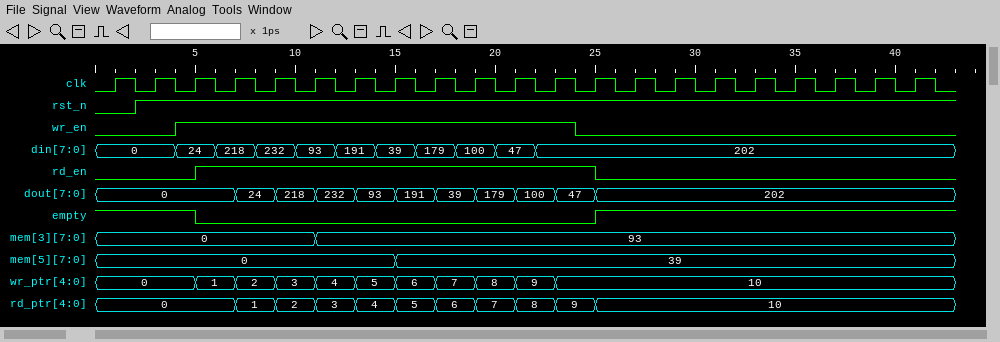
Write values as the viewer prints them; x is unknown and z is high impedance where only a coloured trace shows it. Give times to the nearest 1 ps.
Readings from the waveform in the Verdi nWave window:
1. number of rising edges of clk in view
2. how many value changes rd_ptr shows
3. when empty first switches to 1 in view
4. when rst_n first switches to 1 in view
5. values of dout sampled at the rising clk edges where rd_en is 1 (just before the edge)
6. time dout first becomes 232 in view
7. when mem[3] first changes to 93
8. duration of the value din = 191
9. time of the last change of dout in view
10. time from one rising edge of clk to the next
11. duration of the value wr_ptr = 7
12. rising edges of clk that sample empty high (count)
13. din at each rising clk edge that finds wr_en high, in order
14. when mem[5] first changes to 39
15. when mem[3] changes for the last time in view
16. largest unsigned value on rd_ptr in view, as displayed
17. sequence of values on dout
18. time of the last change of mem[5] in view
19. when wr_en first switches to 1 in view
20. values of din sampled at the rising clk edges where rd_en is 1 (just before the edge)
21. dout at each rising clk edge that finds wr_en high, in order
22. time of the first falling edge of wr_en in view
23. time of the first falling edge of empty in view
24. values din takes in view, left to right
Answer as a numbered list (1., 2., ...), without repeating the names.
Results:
1. 21
2. 10
3. 25 ps
4. 2 ps
5. 0, 24, 218, 232, 93, 191, 39, 179, 100, 47
6. 11 ps
7. 11 ps
8. 2 ps
9. 25 ps
10. 2 ps
11. 2 ps
12. 11
13. 24, 218, 232, 93, 191, 39, 179, 100, 47, 202
14. 15 ps
15. 11 ps
16. 10
17. 0, 24, 218, 232, 93, 191, 39, 179, 100, 47, 202
18. 15 ps
19. 4 ps
20. 218, 232, 93, 191, 39, 179, 100, 47, 202, 202
21. 0, 0, 24, 218, 232, 93, 191, 39, 179, 100
22. 24 ps
23. 5 ps
24. 0, 24, 218, 232, 93, 191, 39, 179, 100, 47, 202
